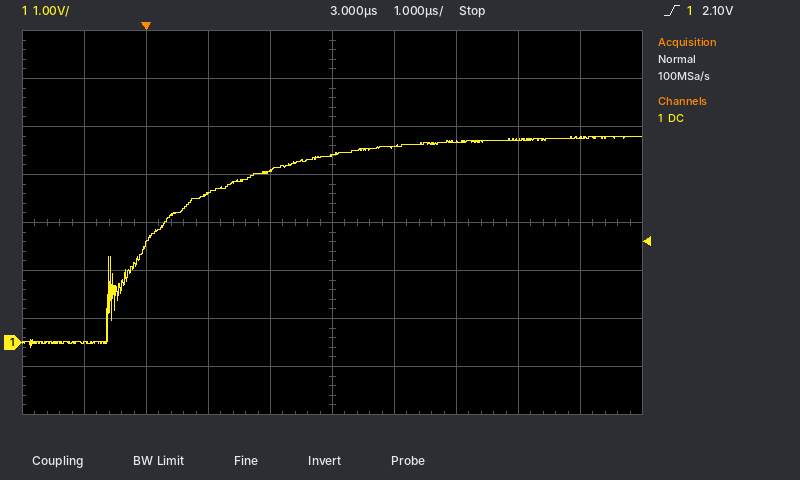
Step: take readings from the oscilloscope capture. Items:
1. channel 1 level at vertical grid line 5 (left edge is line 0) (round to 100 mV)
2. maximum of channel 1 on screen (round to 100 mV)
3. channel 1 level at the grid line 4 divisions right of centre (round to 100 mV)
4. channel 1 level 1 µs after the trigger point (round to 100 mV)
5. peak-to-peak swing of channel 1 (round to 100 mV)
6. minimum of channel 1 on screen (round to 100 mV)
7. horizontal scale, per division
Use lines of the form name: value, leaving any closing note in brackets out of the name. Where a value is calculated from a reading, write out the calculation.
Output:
channel 1 level at vertical grid line 5 (left edge is line 0): 3.9 V
maximum of channel 1 on screen: 4.3 V
channel 1 level at the grid line 4 divisions right of centre: 4.3 V
channel 1 level 1 µs after the trigger point: 3.1 V
peak-to-peak swing of channel 1: 4.3 V − (-100 mV) = 4.4 V
minimum of channel 1 on screen: -100 mV
horizontal scale, per division: 1 µs
